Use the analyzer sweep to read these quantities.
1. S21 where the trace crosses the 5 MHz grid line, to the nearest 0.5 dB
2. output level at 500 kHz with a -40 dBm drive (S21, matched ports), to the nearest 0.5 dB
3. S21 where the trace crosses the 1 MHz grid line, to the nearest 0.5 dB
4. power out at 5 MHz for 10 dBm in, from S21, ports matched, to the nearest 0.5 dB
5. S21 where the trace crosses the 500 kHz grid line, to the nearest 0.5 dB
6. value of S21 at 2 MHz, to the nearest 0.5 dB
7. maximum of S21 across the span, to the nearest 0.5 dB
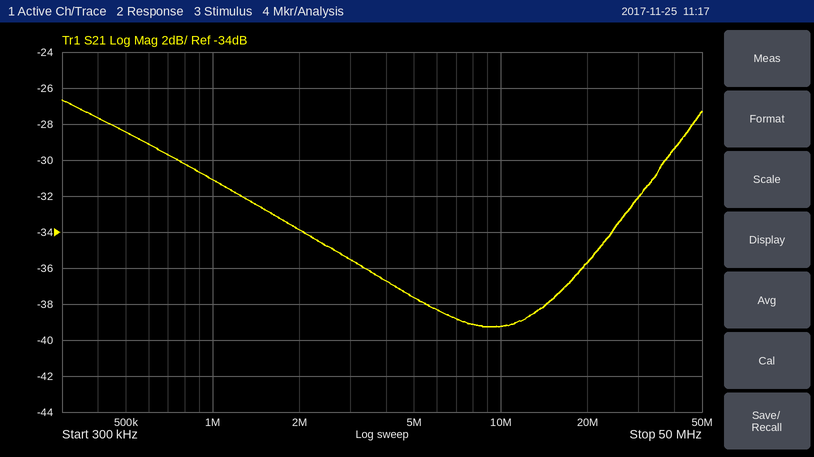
-37.5 dB
-68.5 dBm
-31.0 dB
-27.5 dBm
-28.5 dB
-34.0 dB
-26.5 dB
